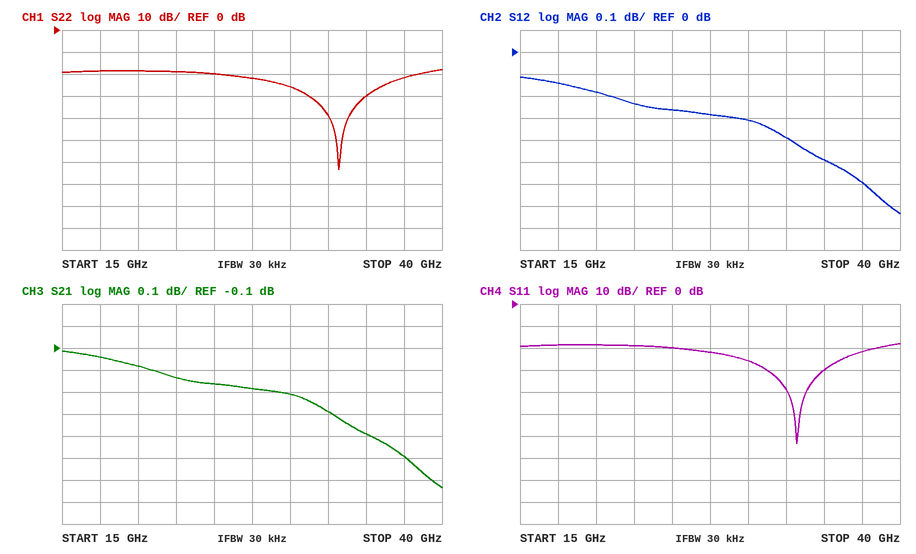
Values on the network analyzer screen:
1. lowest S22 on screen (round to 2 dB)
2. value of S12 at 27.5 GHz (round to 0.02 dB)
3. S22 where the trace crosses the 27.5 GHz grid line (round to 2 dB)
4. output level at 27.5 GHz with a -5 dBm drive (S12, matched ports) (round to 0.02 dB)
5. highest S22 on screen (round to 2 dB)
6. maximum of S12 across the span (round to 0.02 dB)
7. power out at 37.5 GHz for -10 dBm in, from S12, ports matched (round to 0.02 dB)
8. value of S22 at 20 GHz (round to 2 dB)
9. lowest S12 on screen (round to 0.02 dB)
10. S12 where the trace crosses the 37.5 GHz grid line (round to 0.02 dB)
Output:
-64 dB
-0.28 dB
-22 dB
-5.28 dBm
-18 dB
-0.12 dB
-10.60 dBm
-18 dB
-0.74 dB
-0.60 dB
